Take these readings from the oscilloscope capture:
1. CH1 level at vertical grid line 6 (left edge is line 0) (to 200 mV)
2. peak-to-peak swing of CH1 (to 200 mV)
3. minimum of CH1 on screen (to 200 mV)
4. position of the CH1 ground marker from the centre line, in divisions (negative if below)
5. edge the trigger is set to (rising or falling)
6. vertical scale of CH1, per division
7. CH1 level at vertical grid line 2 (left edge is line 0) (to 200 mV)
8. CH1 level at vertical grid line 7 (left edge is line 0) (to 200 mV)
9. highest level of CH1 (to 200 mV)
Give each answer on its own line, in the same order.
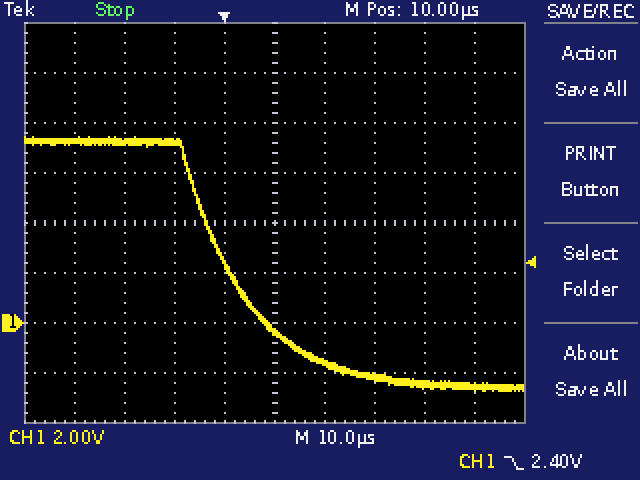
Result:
-1.6 V
10.2 V
-2.8 V
-2.0 div
falling
2 V
7.2 V
-2.2 V
7.4 V
